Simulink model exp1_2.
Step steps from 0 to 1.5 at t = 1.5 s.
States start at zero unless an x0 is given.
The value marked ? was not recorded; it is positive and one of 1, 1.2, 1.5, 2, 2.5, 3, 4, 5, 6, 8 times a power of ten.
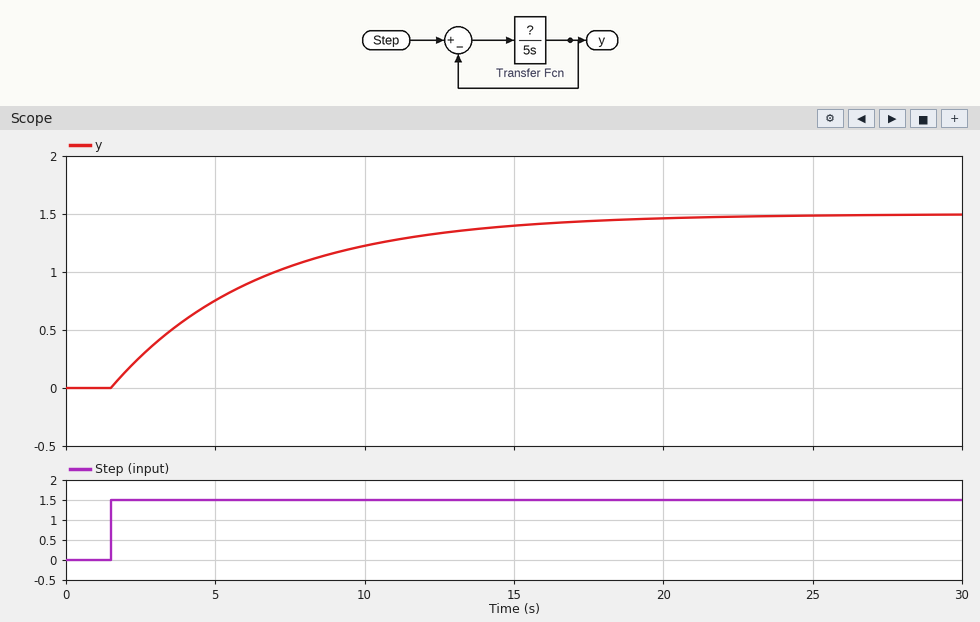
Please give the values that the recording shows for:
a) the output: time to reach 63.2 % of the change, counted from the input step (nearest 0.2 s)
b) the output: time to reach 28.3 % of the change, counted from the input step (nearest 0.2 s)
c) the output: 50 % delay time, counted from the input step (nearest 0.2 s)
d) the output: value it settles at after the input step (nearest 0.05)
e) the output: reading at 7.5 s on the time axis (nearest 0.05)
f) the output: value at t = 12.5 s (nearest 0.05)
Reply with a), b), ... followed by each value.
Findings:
a) 5.0 s
b) 1.6 s
c) 3.4 s
d) 1.50
e) 1.05
f) 1.35
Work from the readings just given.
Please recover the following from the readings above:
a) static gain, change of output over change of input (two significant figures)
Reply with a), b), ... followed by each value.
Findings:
a) 1.0
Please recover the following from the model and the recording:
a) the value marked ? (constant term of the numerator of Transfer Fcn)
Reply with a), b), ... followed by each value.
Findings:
a) 1
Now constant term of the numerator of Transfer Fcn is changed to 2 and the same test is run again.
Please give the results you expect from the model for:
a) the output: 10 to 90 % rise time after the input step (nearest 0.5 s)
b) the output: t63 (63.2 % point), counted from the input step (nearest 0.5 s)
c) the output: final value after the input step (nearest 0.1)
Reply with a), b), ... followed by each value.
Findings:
a) 5.5 s
b) 2.5 s
c) 1.5
